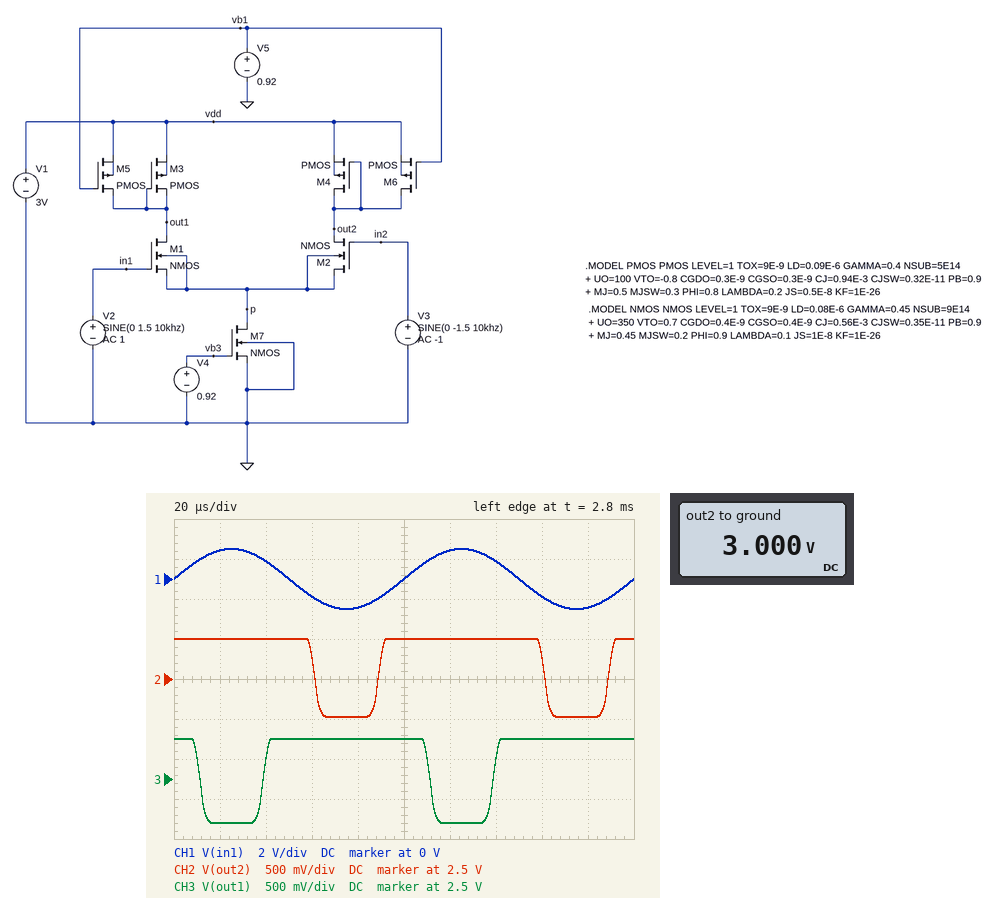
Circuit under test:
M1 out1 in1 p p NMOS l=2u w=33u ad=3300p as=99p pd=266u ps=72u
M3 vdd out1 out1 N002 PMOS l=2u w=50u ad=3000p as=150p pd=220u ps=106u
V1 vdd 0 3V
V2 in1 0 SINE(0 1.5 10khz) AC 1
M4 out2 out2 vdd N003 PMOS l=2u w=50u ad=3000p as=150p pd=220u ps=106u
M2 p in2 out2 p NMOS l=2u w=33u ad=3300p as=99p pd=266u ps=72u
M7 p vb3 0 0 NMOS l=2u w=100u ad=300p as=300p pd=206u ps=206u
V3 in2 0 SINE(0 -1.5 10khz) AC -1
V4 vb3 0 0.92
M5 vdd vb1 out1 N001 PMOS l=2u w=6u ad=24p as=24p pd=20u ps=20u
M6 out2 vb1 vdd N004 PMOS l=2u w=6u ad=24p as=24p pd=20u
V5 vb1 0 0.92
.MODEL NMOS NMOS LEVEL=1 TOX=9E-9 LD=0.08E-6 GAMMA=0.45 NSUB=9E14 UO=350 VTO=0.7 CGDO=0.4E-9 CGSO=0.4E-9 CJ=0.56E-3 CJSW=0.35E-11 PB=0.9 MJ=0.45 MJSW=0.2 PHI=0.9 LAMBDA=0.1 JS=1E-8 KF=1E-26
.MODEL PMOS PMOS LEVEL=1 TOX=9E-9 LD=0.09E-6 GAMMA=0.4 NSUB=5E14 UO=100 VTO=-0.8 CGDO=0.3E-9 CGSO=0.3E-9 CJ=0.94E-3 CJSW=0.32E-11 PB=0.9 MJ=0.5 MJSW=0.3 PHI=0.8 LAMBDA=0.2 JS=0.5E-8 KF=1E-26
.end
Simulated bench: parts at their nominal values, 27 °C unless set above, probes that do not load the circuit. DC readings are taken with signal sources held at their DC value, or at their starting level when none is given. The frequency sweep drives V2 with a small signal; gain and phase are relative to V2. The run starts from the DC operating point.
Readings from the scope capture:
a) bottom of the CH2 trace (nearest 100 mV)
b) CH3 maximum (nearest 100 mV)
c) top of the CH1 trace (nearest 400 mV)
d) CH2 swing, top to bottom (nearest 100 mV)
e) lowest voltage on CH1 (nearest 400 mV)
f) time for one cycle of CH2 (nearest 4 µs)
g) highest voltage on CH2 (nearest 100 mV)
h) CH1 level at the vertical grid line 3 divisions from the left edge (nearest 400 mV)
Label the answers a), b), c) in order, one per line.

a) 2.0 V
b) 3.0 V
c) 1.6 V
d) 1.0 V
e) -1.6 V
f) 100 µs
g) 3.0 V
h) -800 mV
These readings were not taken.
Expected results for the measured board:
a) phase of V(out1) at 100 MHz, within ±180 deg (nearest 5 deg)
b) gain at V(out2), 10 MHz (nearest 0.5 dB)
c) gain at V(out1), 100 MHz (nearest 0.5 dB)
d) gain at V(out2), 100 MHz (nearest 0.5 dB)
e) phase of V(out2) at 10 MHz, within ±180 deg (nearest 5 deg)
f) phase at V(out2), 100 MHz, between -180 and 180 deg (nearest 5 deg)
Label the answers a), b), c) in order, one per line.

a) 20 deg
b) -46.0 dB
c) -40.0 dB
d) -28.5 dB
e) -95 deg
f) -130 deg
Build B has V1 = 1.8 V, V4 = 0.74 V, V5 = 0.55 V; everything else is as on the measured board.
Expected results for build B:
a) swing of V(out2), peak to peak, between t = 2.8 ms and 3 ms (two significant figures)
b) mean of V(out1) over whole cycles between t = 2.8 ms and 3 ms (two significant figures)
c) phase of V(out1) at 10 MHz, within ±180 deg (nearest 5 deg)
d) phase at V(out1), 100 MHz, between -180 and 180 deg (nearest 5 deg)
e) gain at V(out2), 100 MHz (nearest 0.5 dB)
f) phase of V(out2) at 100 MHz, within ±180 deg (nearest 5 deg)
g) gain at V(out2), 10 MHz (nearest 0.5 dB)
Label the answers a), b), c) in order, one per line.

a) 120 mV
b) 1.8 V
c) 35 deg
d) 10 deg
e) -25.5 dB
f) -160 deg
g) -37.0 dB
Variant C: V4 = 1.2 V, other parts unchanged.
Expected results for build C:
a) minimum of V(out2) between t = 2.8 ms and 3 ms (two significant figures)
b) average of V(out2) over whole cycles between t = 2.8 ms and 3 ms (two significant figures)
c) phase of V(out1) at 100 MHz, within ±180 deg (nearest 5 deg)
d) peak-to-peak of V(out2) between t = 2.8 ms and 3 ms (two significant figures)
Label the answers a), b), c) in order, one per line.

a) 1.6 V
b) 2.6 V
c) 15 deg
d) 1.4 V
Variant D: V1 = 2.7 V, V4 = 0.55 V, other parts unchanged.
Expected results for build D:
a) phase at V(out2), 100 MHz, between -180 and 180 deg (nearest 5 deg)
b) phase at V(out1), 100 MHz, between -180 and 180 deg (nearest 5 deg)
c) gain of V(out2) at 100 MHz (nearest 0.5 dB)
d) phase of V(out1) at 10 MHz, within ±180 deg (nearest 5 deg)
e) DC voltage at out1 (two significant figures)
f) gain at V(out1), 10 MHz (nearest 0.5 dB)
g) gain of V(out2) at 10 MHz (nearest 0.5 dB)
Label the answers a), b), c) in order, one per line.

a) -140 deg
b) 10 deg
c) -27.5 dB
d) 65 deg
e) 2.7 V
f) -44.5 dB
g) -43.5 dB
